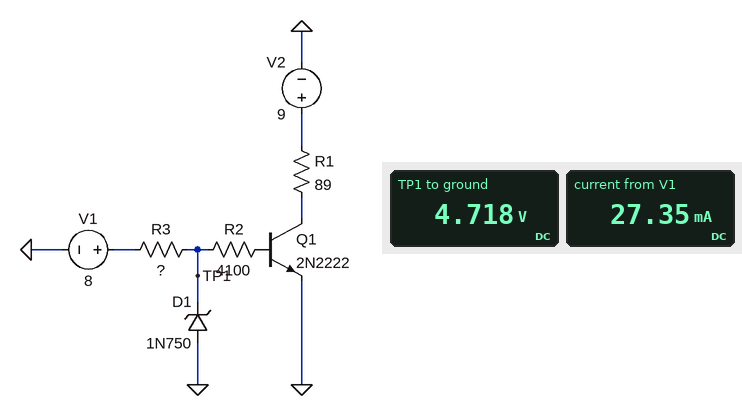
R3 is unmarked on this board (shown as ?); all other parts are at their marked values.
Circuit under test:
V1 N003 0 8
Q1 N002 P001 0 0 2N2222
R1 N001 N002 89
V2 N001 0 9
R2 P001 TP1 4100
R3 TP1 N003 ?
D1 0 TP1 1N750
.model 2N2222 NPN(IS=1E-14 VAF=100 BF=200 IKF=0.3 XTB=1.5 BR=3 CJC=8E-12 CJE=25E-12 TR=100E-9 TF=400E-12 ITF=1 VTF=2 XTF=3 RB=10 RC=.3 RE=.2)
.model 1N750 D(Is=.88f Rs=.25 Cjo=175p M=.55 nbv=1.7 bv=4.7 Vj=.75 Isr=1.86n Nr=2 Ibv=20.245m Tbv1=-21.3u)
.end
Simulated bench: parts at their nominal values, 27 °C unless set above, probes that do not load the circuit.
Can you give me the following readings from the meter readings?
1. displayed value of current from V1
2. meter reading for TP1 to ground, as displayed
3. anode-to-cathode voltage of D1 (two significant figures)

27.35 mA
4.718 V
-4.7 V
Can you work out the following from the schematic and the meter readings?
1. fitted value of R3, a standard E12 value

120 Ω
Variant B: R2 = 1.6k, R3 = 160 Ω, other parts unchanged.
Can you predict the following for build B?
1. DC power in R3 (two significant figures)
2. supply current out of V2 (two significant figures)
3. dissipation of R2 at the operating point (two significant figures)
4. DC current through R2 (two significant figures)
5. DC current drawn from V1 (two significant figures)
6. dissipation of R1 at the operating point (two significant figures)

68 mW
100 mA
9.4 mW
2.4 mA
21 mA
880 mW
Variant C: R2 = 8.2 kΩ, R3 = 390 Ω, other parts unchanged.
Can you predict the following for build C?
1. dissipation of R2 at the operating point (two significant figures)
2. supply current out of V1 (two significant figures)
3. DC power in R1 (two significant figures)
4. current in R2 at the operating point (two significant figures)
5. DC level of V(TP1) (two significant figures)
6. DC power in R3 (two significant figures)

1.8 mW
8.6 mA
520 mW
470 µA
4.7 V
29 mW
